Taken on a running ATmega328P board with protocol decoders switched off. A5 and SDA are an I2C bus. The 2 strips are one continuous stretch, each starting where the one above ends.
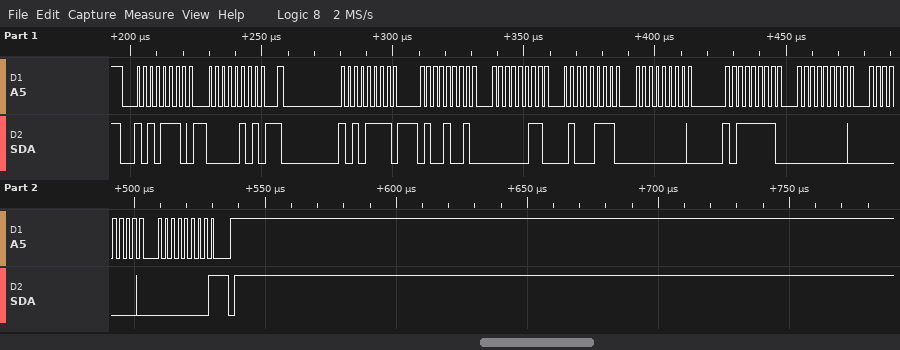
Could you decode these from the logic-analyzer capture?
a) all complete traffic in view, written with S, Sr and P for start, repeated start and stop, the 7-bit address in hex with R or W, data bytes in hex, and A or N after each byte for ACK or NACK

S 57W A 05 A Sr 57R A 49 A 03 A 47 A 00 A BF A 00 A 00 A 00 N P
